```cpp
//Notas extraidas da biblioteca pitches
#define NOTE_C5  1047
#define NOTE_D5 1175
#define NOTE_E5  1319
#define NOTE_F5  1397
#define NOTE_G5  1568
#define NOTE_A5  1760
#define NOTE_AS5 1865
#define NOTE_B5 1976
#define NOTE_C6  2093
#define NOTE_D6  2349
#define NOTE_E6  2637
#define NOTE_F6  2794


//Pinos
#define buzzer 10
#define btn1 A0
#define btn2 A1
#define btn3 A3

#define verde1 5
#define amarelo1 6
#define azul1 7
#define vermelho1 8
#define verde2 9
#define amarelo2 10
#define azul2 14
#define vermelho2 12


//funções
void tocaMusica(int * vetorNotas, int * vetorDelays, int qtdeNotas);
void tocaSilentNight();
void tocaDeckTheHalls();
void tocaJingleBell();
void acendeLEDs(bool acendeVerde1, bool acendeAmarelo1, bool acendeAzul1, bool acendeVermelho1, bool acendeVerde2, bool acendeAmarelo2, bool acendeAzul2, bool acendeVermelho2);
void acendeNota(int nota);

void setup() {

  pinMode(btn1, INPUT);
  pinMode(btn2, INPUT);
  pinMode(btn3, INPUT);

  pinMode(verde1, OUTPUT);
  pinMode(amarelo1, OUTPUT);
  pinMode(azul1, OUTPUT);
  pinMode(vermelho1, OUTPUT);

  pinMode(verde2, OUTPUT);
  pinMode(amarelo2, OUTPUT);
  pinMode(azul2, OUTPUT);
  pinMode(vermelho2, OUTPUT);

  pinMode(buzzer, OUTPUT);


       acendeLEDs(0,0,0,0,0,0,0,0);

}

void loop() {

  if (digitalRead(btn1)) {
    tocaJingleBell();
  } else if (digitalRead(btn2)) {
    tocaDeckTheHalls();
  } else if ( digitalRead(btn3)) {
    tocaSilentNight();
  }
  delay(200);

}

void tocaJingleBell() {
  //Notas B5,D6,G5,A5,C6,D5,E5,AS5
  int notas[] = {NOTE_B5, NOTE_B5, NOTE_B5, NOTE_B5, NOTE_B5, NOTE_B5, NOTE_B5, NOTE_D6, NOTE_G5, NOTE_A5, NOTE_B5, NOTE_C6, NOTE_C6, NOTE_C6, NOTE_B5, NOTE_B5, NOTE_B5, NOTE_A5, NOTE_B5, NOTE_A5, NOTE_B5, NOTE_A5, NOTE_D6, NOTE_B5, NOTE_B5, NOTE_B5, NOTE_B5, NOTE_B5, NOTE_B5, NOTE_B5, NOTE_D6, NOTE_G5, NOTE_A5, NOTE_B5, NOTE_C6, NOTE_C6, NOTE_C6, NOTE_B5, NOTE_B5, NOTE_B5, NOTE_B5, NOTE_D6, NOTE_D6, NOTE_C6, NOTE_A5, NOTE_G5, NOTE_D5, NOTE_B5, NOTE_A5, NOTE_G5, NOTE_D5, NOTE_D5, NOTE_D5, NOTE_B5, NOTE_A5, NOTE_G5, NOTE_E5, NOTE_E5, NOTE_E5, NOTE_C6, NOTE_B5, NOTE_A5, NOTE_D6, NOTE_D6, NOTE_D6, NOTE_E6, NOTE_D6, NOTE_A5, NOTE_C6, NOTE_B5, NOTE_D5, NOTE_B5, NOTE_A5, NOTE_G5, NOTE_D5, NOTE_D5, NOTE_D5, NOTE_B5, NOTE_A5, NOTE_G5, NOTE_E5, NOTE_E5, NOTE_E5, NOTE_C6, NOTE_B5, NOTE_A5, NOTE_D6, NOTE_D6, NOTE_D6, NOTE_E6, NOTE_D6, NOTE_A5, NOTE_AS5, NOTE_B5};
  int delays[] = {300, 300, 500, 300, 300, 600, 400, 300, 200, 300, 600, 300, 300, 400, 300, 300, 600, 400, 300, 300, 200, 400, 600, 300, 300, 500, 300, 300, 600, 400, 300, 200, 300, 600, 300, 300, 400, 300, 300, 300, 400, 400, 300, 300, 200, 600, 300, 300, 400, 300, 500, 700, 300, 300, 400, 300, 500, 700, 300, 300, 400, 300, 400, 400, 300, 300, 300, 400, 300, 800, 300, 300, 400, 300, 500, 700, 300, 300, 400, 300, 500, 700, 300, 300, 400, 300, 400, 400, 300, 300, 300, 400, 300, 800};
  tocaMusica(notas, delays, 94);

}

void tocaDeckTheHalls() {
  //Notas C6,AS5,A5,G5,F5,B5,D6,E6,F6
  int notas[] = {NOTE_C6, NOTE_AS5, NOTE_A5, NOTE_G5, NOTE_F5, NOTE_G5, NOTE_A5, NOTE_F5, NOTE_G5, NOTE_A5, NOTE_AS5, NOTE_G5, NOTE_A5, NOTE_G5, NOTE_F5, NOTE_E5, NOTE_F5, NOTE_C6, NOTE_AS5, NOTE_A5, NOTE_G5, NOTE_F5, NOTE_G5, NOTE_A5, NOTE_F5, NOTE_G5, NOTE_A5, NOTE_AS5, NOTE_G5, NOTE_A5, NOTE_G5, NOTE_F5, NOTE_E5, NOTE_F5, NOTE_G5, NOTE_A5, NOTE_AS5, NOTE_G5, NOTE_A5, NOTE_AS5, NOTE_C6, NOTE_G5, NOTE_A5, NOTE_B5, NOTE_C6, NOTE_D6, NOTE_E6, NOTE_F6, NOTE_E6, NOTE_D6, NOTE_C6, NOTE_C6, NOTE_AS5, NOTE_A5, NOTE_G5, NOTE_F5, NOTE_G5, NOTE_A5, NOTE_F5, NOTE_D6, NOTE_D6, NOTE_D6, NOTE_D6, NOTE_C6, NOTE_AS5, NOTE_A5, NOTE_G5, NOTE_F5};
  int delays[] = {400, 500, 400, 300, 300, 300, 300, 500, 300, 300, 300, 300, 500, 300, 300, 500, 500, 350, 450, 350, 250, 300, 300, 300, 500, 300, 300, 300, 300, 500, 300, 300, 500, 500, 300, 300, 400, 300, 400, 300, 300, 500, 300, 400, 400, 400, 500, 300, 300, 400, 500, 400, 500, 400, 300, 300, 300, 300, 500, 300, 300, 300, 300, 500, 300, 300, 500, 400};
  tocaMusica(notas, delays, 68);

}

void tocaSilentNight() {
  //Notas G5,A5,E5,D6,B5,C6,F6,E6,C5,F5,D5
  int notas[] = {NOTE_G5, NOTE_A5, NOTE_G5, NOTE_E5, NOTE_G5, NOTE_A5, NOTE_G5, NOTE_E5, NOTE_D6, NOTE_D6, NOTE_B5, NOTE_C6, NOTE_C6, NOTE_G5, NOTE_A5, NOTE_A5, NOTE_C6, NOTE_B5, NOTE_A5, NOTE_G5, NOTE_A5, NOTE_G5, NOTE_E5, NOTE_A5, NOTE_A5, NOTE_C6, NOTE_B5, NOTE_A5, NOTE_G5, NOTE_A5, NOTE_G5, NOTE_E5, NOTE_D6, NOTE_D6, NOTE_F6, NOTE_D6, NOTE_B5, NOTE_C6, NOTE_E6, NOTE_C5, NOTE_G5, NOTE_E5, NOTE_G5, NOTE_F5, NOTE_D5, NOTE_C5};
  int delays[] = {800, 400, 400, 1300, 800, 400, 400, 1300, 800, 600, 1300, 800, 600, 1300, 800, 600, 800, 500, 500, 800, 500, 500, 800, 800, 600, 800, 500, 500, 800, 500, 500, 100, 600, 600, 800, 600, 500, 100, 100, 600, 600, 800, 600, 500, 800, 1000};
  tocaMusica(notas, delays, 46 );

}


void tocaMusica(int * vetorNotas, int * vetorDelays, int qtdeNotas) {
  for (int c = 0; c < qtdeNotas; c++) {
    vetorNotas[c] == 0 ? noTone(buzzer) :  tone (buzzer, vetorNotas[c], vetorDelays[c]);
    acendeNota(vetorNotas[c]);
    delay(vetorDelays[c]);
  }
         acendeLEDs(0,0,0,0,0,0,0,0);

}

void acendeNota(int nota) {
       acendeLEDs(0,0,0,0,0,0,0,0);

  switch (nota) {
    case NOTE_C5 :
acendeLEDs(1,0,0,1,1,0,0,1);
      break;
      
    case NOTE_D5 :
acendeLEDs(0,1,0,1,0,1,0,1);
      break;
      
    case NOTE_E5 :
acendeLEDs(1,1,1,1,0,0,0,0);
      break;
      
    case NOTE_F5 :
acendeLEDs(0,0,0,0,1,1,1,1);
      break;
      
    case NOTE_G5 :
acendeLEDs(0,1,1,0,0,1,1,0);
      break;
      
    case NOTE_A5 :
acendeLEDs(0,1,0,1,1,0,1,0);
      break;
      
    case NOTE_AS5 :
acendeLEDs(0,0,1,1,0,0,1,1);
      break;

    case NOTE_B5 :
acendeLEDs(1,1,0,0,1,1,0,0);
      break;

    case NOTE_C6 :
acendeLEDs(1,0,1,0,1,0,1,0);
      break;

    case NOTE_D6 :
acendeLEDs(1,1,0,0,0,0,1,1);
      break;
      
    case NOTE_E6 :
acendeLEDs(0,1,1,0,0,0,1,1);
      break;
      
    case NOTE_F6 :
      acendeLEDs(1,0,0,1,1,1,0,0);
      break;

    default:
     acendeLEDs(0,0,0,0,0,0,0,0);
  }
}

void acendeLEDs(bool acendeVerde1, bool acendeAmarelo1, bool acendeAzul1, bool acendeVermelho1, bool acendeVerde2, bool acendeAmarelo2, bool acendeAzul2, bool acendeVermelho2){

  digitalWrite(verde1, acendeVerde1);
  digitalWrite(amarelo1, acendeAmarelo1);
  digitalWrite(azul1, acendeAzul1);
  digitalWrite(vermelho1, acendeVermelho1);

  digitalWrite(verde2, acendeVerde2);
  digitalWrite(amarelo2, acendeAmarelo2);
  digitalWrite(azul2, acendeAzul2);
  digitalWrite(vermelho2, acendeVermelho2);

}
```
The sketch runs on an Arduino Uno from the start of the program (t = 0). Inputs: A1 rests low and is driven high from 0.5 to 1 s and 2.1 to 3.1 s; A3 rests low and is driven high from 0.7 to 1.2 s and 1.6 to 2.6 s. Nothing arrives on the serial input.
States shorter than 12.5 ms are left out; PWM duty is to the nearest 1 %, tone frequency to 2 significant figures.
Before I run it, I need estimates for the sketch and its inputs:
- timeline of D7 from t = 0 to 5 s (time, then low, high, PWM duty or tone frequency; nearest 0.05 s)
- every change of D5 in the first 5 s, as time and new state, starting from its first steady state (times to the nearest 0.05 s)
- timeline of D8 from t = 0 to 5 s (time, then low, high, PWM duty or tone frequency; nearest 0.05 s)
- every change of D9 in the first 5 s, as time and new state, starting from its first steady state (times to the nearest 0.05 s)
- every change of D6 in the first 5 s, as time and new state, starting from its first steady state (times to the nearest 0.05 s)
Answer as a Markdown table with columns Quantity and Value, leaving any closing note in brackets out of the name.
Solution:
| Quantity | Value |
|---|---|
| timeline of D7 from t = 0 to 5 s | 0 s low; 0.6 s high; 1.5 s low; 1.9 s high; 2.2 s low; 2.5 s high; 2.8 s low; 3.6 s high; 3.9 s low; 4.2 s high; 4.8 s low |
| every change of D5 in the first 5 s, as time and new state, starting from its first steady state | 0 s low; 0.6 s high; 1 s low |
| timeline of D8 from t = 0 to 5 s | 0 s low; 1 s high; 1.9 s low; 2.8 s high; 3.1 s low; 3.9 s high; 4.5 s low; 4.8 s high |
| every change of D9 in the first 5 s, as time and new state, starting from its first steady state | 0 s low; 0.6 s high; 1 s low; 1.5 s high; 1.9 s low; 2.2 s high; 2.5 s low; 2.8 s high; 3.6 s low; 3.9 s high; 4.2 s low; 4.8 s high |
| every change of D6 in the first 5 s, as time and new state, starting from its first steady state | 0 s low; 1.5 s high; 2.2 s low; 2.5 s high; 3.1 s low; 3.6 s high; 4.2 s low; 4.5 s high |
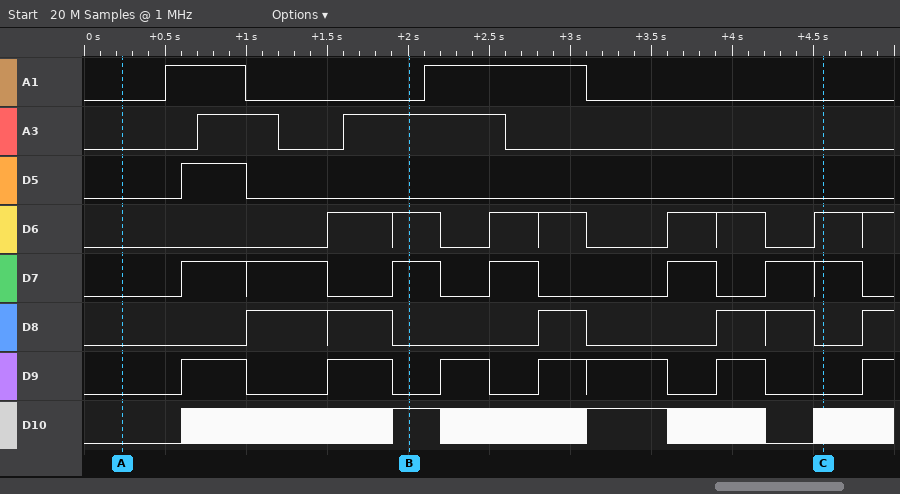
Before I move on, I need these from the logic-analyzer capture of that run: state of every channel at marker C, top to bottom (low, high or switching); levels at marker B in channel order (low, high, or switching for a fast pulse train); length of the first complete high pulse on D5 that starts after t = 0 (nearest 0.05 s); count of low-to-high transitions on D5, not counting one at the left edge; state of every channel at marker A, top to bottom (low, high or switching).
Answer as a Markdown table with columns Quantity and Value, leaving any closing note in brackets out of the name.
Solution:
| Quantity | Value |
|---|---|
| state of every channel at marker C, top to bottom | A1 low, A3 low, D5 low, D6 high, D7 high, D8 low, D9 low, D10 switching |
| levels at marker B in channel order | A1 low, A3 high, D5 low, D6 high, D7 high, D8 low, D9 low, D10 high |
| length of the first complete high pulse on D5 that starts after t = 0 | 0.40 s |
| count of low-to-high transitions on D5, not counting one at the left edge | 1 |
| state of every channel at marker A, top to bottom | A1 low, A3 low, D5 low, D6 low, D7 low, D8 low, D9 low, D10 low |
